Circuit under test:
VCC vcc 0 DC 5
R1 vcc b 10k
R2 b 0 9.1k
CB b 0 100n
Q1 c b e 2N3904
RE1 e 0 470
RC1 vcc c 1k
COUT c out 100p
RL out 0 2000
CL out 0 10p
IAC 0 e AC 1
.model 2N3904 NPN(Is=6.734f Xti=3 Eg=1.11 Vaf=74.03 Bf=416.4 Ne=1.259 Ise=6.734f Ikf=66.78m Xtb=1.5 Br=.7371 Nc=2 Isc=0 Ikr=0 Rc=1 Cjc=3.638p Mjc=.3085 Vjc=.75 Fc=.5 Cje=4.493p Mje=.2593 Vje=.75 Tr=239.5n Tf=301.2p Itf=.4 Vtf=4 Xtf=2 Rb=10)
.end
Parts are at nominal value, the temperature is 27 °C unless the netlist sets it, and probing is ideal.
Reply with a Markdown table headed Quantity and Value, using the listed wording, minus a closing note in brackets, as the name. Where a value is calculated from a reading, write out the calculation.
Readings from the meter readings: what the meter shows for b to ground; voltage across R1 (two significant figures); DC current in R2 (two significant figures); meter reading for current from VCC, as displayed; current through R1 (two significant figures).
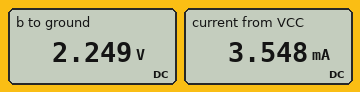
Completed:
| Quantity | Value |
|---|---|
| what the meter shows for b to ground | 2.249 V |
| voltage across R1 | 5 V - 2.249 V = 2.8 V |
| DC current in R2 | (2.249 V) / 9.1 kΩ = 250 µA |
| meter reading for current from VCC, as displayed | 3.548 mA |
| current through R1 | (5 V - 2.249 V) / 10 kΩ = 280 µA |
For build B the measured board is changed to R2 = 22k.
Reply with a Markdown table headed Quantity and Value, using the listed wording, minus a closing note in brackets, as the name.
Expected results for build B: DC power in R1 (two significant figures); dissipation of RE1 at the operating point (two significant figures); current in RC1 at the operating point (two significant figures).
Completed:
| Quantity | Value |
|---|---|
| DC power in R1 | 720 µW |
| dissipation of RE1 at the operating point | 5.6 mW |
| current in RC1 at the operating point | 3.3 mA |
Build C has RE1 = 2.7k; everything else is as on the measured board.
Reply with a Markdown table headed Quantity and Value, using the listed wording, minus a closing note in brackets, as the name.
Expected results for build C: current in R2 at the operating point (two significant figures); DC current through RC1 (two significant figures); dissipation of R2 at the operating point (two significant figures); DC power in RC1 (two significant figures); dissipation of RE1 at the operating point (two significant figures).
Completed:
| Quantity | Value |
|---|---|
| current in R2 at the operating point | 260 µA |
| DC current through RC1 | 630 µA |
| dissipation of R2 at the operating point | 610 µW |
| DC power in RC1 | 390 µW |
| dissipation of RE1 at the operating point | 1.1 mW |
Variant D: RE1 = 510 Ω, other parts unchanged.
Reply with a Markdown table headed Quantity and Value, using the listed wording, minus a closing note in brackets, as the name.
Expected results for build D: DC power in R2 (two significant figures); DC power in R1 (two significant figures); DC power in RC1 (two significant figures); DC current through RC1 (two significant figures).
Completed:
| Quantity | Value |
|---|---|
| DC power in R2 | 570 µW |
| DC power in R1 | 740 µW |
| DC power in RC1 | 9.6 mW |
| DC current through RC1 | 3.1 mA |
